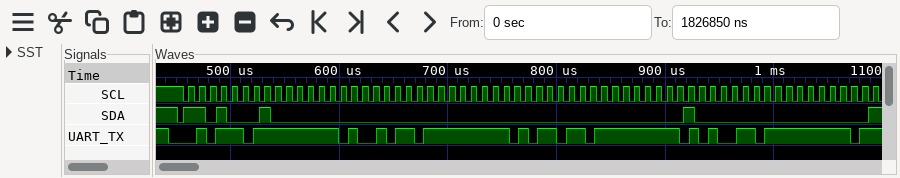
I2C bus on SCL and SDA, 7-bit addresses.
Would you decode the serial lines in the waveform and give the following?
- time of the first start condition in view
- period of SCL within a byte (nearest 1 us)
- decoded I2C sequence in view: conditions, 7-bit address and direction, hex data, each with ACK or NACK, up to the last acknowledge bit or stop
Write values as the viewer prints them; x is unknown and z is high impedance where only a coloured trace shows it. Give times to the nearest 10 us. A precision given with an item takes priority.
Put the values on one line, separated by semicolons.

450 us; 10 us; start, address 68 read ACK, 00 ACK, 00 ACK, 00 ACK, 00 ACK, 40 ACK, 00 ACK
